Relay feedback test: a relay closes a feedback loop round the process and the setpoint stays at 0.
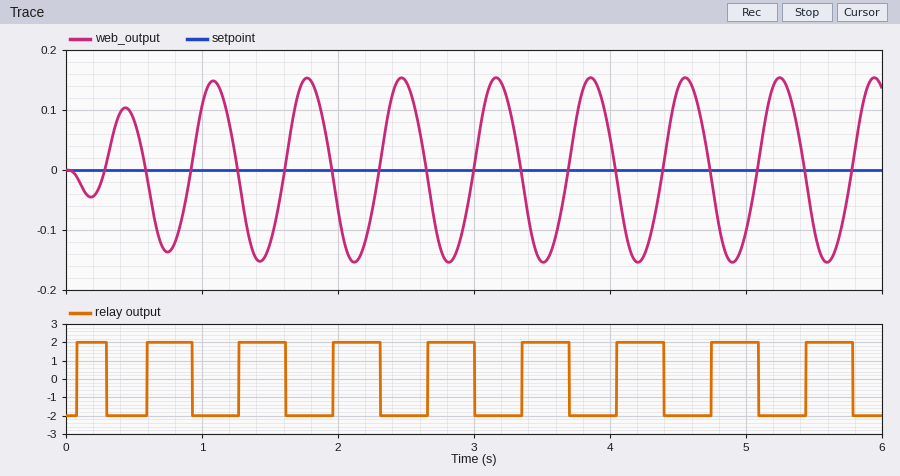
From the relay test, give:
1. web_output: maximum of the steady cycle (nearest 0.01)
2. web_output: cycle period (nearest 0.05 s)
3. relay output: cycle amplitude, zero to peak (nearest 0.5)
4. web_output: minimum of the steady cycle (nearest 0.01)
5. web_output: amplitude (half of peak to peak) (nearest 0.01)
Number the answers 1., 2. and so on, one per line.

1. 0.15
2. 0.70 s
3. 2.0
4. -0.15
5. 0.15
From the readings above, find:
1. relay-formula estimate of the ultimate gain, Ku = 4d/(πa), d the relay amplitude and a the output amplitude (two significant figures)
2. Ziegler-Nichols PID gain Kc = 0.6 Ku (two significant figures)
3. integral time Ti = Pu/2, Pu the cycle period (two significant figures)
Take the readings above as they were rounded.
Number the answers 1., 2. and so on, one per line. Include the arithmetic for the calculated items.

1. 4 × 2 / (π × 0.15) = 17
2. 0.6 × 17 = 10
3. 0.7 / 2 = 0.35 s
